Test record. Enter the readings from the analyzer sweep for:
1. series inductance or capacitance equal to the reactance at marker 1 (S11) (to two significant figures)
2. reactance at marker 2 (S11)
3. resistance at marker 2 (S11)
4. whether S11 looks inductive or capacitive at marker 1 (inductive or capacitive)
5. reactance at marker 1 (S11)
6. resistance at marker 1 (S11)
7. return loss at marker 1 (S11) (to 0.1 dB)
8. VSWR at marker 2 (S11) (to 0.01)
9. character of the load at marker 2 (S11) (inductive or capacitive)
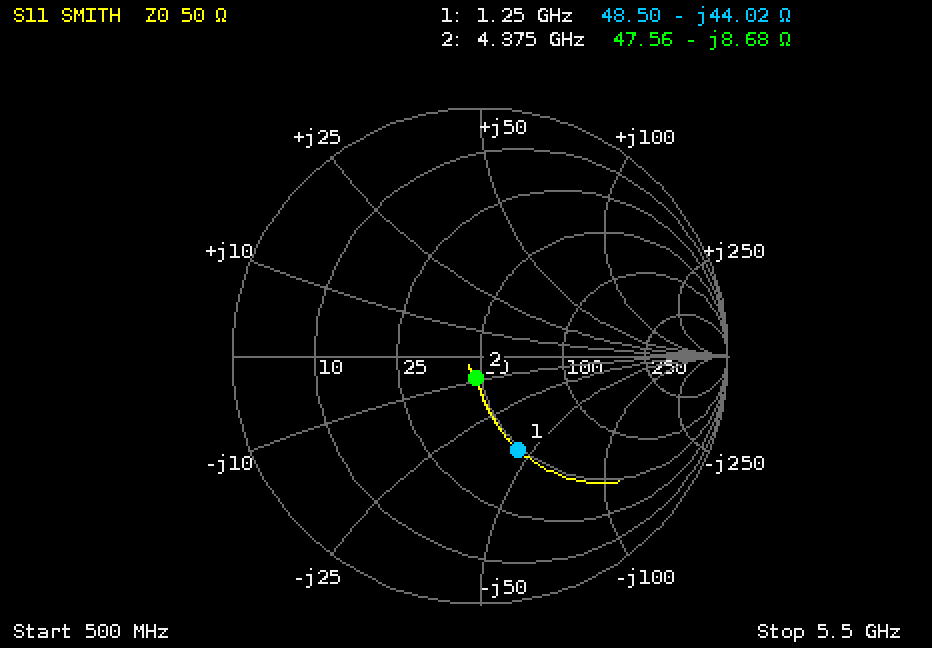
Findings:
2.9 pF
-8.68 Ω
47.56 Ω
capacitive
-44.02 Ω
48.50 Ω
7.8 dB
1.20
capacitive
